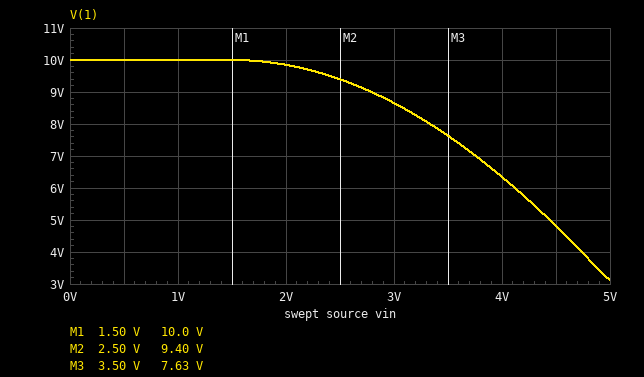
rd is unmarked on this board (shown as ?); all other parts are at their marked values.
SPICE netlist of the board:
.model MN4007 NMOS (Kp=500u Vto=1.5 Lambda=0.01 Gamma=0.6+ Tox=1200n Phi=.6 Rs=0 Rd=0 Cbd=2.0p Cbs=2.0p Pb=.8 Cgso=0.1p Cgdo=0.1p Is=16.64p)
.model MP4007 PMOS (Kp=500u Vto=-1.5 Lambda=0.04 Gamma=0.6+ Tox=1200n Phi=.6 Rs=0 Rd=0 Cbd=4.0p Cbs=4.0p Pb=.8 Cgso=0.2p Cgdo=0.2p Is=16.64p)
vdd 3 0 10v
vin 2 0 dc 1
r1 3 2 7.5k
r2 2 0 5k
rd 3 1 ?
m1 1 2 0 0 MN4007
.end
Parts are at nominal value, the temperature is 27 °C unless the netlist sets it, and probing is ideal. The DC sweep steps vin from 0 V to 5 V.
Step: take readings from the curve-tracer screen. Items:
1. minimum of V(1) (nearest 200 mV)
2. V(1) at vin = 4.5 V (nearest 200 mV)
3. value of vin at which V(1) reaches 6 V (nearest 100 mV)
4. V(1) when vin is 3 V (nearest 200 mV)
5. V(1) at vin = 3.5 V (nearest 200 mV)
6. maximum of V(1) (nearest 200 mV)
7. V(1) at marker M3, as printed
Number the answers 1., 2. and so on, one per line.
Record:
1. 3.2 V
2. 4.8 V
3. 4.1 V
4. 8.6 V
5. 7.6 V
6. 10.0 V
7. 7.63 V
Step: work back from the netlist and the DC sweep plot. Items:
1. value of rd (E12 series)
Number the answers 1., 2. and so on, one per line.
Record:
1. 2.2 kΩ
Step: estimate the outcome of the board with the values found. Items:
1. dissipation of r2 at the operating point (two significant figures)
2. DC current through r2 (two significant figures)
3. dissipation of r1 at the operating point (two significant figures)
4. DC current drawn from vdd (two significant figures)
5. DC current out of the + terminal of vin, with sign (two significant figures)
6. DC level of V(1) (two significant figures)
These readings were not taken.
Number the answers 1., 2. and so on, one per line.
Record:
1. 200 µW
2. 200 µA
3. 11 mW
4. 1.2 mA
5. -1.0 mA
6. 10 V
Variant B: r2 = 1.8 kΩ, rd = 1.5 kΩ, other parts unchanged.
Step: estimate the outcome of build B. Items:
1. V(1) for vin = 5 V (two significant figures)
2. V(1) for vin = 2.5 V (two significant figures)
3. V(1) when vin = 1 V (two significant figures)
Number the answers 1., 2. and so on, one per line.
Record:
1. 5.2 V
2. 9.6 V
3. 10 V
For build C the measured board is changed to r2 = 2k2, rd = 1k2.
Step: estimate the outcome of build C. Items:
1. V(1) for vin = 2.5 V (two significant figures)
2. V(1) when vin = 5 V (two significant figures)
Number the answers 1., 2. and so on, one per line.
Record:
1. 9.7 V
2. 6.1 V
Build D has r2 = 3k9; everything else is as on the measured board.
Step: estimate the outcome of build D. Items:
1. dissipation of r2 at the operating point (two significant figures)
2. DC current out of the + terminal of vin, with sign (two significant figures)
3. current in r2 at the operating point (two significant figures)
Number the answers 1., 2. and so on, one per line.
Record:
1. 260 µW
2. -940 µA
3. 260 µA
